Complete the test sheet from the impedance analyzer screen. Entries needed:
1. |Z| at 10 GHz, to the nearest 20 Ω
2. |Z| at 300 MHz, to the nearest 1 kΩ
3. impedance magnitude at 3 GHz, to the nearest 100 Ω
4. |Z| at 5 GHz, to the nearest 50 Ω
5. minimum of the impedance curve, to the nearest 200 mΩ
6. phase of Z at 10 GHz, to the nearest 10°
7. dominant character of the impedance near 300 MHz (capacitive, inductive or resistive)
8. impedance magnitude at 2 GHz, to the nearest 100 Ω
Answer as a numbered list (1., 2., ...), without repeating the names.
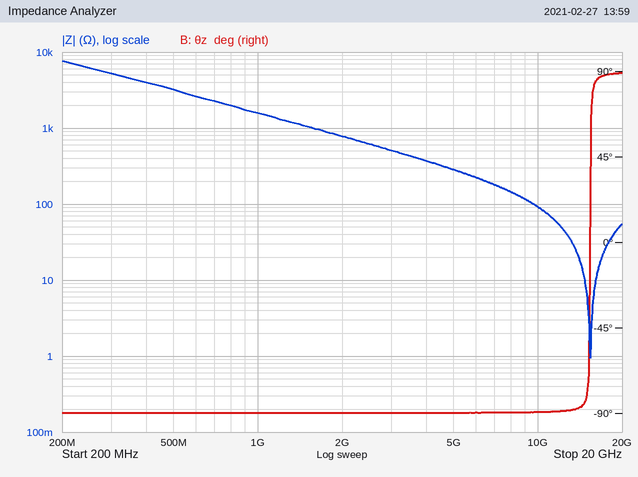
1. 100 Ω
2. 5 kΩ
3. 500 Ω
4. 300 Ω
5. 1.0 Ω
6. -90°
7. capacitive
8. 800 Ω
